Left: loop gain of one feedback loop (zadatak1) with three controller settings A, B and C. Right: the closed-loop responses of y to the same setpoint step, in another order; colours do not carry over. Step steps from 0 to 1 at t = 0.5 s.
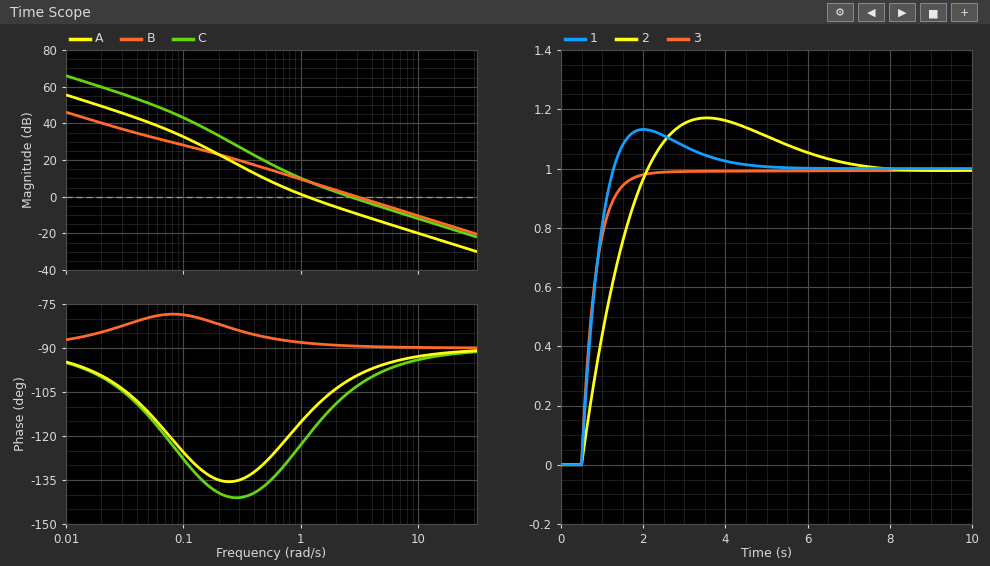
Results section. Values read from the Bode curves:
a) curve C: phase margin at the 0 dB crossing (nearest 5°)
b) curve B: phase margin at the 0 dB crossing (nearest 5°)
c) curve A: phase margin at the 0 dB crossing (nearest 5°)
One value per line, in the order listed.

75°
90°
65°
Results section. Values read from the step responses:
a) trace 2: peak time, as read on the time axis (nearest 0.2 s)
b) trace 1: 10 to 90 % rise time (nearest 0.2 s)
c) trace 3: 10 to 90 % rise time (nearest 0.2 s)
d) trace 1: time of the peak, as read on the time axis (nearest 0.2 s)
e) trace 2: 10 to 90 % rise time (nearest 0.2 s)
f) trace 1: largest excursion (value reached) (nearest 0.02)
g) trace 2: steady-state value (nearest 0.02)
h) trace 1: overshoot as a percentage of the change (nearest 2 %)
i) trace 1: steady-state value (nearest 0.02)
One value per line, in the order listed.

3.6 s
0.6 s
0.8 s
2.0 s
1.2 s
1.14
1.00
14 %
1.00
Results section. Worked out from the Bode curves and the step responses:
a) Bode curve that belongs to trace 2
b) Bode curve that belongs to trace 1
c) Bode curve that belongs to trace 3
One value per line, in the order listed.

A
C
B
